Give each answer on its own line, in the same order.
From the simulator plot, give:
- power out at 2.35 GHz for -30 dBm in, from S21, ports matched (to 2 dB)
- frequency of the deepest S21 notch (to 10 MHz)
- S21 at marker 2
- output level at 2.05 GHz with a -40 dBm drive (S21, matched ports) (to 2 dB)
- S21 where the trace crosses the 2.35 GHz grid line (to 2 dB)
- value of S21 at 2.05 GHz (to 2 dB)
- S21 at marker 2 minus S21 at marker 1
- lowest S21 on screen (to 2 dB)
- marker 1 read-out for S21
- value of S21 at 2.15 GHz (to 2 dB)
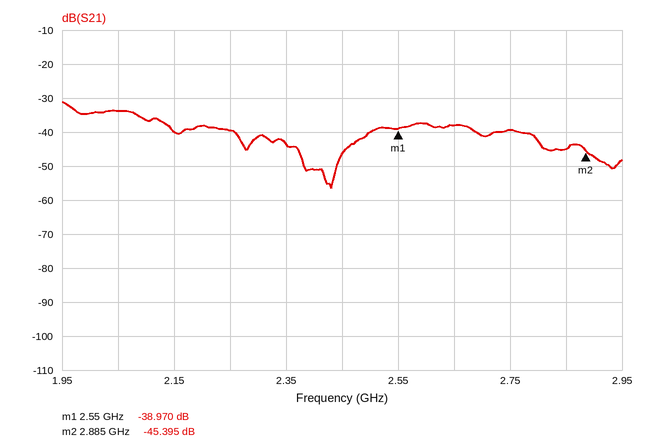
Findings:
-74 dBm
2.43 GHz
-45.395 dB
-74 dBm
-44 dB
-34 dB
-6.425 dB
-56 dB
-38.970 dB
-40 dB
